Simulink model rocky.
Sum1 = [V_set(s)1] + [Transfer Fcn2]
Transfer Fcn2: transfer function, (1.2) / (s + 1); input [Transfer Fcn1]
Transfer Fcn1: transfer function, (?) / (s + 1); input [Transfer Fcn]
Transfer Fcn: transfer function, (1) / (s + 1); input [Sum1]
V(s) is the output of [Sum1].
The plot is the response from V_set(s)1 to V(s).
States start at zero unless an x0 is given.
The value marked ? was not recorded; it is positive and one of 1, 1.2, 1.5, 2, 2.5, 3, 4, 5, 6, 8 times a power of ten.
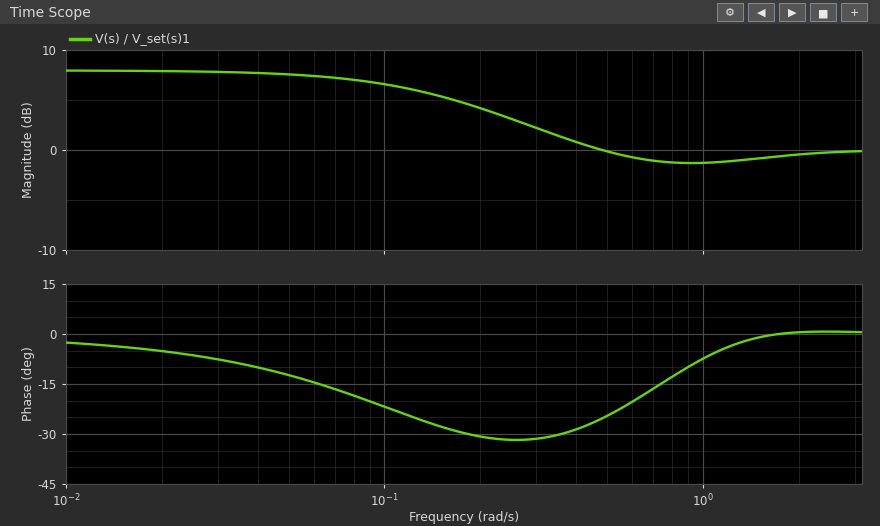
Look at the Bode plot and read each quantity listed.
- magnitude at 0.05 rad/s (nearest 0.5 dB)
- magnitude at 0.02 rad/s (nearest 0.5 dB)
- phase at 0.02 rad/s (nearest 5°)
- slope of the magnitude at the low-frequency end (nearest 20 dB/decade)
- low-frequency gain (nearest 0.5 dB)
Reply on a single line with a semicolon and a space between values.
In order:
7.5 dB; 8.0 dB; -5°; 0 dB/decade; 8.0 dB
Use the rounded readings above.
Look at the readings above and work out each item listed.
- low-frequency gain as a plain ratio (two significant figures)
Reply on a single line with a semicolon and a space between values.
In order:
2.5
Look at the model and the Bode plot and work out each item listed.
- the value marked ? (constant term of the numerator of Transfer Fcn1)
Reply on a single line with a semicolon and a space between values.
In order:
0.5
